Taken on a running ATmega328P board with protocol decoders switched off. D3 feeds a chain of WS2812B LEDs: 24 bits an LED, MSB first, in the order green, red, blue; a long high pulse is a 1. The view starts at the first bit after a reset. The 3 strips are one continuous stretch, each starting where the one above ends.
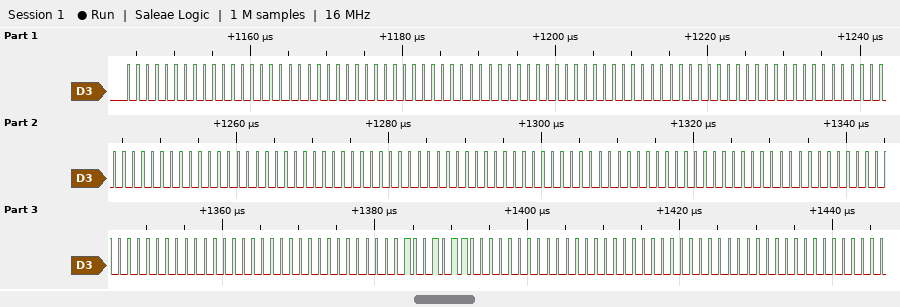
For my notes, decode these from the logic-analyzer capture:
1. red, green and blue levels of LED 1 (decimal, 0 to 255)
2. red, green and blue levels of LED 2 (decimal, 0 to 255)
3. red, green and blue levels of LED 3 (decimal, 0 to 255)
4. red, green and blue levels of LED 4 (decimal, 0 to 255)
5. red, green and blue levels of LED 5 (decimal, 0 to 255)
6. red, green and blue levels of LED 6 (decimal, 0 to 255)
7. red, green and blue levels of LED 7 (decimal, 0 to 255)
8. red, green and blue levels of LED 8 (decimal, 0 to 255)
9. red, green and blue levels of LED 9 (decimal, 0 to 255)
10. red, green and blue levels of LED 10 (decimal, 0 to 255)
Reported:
0, 0, 0
0, 0, 0
0, 0, 0
0, 0, 0
0, 0, 0
0, 0, 0
0, 0, 0
0, 0, 0
0, 150, 0
0, 0, 0
